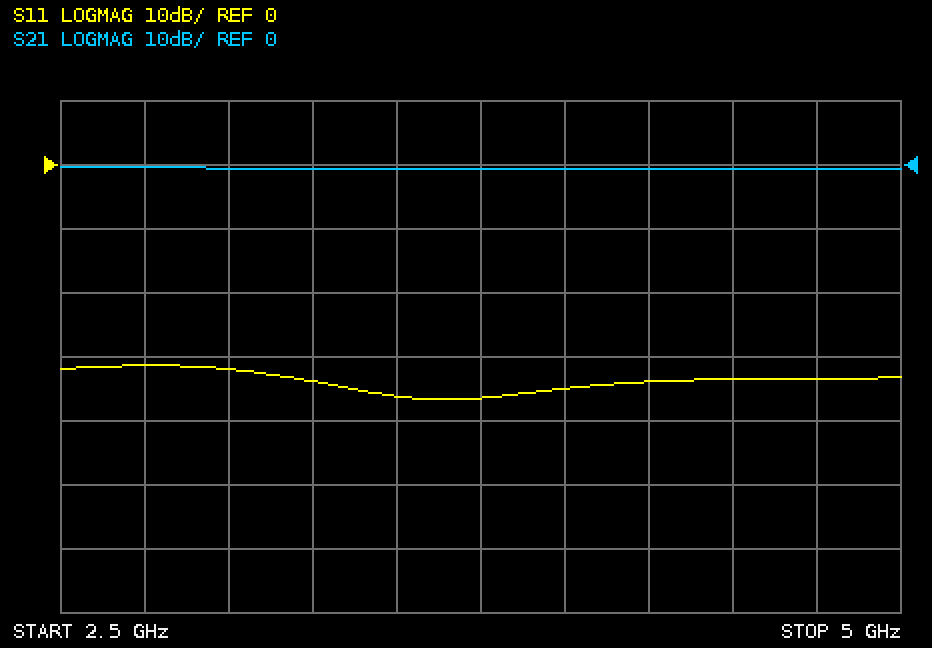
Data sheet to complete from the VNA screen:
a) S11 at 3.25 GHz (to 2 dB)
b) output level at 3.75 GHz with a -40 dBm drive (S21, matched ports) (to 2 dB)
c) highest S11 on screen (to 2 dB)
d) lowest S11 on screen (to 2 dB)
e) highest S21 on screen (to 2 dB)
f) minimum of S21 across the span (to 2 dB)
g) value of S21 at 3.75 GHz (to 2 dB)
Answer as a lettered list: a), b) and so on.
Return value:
a) -34 dB
b) -40 dBm
c) -32 dB
d) -36 dB
e) 0 dB
f) 0 dB
g) 0 dB
